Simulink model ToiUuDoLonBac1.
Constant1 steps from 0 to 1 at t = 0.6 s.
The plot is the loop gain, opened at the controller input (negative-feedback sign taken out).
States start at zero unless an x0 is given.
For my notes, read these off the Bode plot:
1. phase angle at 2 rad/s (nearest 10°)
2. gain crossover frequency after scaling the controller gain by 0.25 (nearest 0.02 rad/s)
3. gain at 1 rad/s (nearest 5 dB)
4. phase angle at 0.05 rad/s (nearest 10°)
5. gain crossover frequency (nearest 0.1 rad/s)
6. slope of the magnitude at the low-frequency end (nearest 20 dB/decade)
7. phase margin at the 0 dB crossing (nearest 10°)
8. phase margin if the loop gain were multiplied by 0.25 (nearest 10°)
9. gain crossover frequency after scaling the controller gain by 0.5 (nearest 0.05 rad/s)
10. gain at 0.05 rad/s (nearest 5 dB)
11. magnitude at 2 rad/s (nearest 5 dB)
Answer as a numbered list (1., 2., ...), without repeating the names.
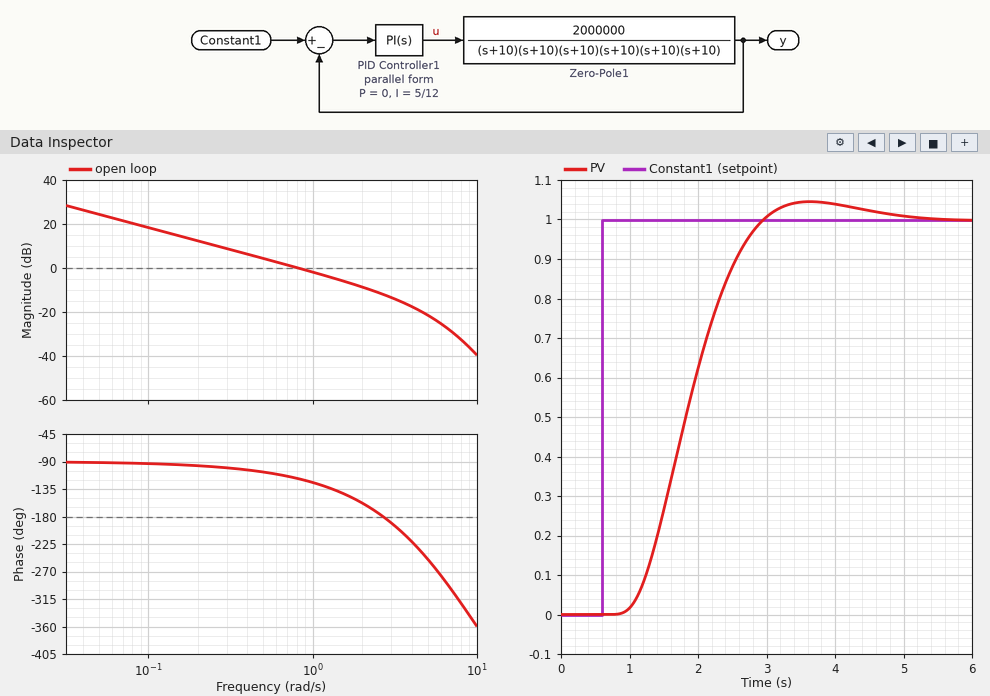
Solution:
1. -160°
2. 0.20 rad/s
3. 0 dB
4. -90°
5. 0.8 rad/s
6. -20 dB/decade
7. 60°
8. 80°
9. 0.40 rad/s
10. 25 dB
11. -10 dB
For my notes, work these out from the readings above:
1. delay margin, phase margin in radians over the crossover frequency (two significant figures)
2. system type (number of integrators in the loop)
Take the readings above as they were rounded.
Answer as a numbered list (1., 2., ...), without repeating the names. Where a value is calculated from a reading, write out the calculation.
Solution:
1. 60 × π / 180 / 0.8 = 1.3 s
2. 1
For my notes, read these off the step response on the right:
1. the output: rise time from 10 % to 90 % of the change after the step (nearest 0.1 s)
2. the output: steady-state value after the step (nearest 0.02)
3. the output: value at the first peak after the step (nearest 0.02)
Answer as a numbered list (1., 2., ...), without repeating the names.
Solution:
1. 1.3 s
2. 1.00
3. 1.04
